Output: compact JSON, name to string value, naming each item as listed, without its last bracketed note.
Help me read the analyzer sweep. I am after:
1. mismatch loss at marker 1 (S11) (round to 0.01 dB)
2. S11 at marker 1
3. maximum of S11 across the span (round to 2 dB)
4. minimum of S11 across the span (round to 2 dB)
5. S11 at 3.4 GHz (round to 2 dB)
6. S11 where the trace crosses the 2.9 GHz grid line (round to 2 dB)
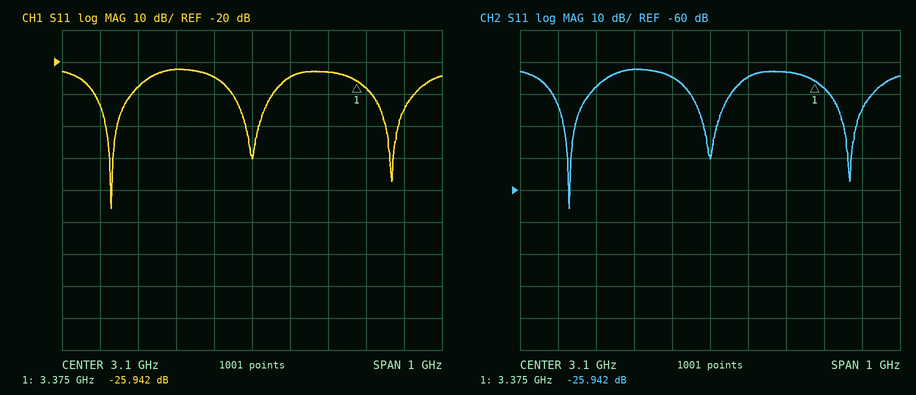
{"mismatch loss at marker 1 (S11)": "0.01 dB", "S11 at marker 1": "-25.942 dB", "maximum of S11 across the span": "-22 dB", "minimum of S11 across the span": "-66 dB", "S11 at 3.4 GHz": "-28 dB", "S11 where the trace crosses the 2.9 GHz grid line": "-22 dB"}
